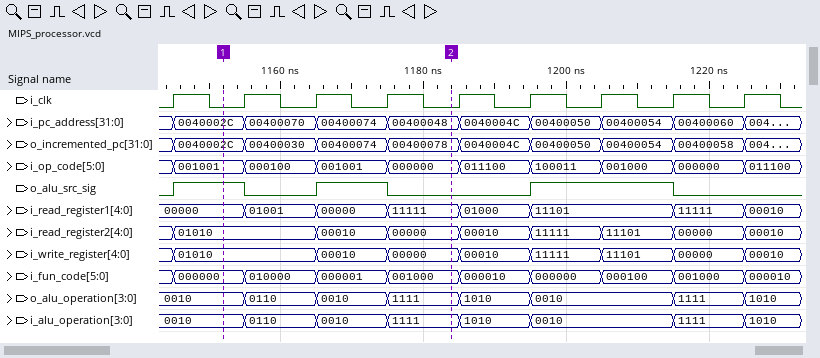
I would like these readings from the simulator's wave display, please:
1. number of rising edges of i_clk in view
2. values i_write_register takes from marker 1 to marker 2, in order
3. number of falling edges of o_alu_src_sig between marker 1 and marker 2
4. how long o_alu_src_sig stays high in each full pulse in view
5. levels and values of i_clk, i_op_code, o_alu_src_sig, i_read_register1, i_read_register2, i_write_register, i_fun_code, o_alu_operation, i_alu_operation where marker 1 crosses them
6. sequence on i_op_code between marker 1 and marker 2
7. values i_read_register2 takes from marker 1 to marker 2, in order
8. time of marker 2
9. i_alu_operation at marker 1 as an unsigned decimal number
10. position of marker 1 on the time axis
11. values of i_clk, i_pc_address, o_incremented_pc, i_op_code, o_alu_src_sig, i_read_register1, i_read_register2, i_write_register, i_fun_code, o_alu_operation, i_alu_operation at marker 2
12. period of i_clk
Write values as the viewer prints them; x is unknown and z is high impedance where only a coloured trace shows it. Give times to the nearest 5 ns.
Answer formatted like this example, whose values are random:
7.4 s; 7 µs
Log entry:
9; 01010, 00010, 00000; 2; 10 ns, 10 ns, 20 ns; i_clk=0, i_op_code=001001, o_alu_src_sig=1, i_read_register1=00000, i_read_register2=01010, i_write_register=01010, i_fun_code=000000, o_alu_operation=0010, i_alu_operation=0010; 001001, 000100, 001001, 000000; 01010, 00010, 00000; 1185 ns; 2; 1150 ns; i_clk=0, i_pc_address=00400048, o_incremented_pc=00400078, i_op_code=000000, o_alu_src_sig=0, i_read_register1=11111, i_read_register2=00000, i_write_register=00000, i_fun_code=001000, o_alu_operation=1111, i_alu_operation=1111; 10 ns
